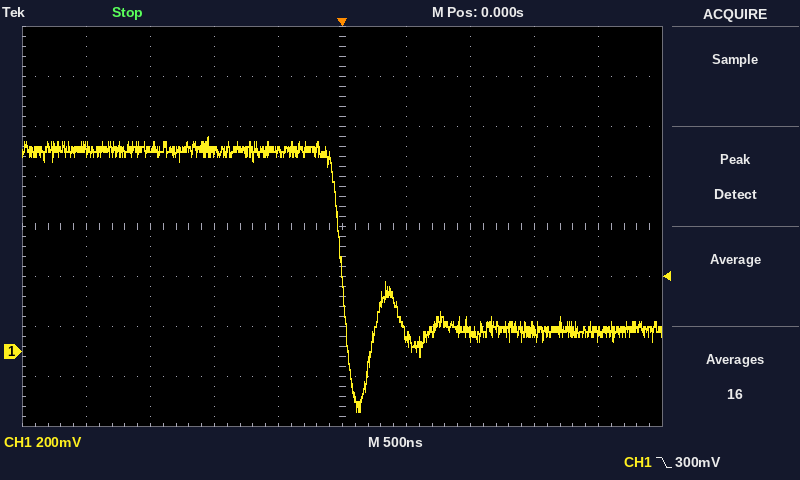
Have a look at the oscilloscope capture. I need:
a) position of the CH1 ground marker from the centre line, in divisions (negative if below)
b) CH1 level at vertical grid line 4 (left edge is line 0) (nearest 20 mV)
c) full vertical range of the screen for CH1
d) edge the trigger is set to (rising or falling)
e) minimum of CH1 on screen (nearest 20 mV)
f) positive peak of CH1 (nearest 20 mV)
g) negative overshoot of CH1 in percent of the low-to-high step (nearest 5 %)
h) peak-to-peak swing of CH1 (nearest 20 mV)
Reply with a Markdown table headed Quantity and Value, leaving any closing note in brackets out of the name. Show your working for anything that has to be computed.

| Quantity | Value |
|---|---|
| position of the CH1 ground marker from the centre line, in divisions | -2.5 div |
| CH1 level at vertical grid line 4 (left edge is line 0) | 800 mV |
| full vertical range of the screen for CH1 | 1.6 V |
| edge the trigger is set to | falling |
| minimum of CH1 on screen | -240 mV |
| positive peak of CH1 | 860 mV |
| negative overshoot of CH1 in percent of the low-to-high step | 45 % |
| peak-to-peak swing of CH1 | 860 mV − (-240 mV) = 1.10 V |
